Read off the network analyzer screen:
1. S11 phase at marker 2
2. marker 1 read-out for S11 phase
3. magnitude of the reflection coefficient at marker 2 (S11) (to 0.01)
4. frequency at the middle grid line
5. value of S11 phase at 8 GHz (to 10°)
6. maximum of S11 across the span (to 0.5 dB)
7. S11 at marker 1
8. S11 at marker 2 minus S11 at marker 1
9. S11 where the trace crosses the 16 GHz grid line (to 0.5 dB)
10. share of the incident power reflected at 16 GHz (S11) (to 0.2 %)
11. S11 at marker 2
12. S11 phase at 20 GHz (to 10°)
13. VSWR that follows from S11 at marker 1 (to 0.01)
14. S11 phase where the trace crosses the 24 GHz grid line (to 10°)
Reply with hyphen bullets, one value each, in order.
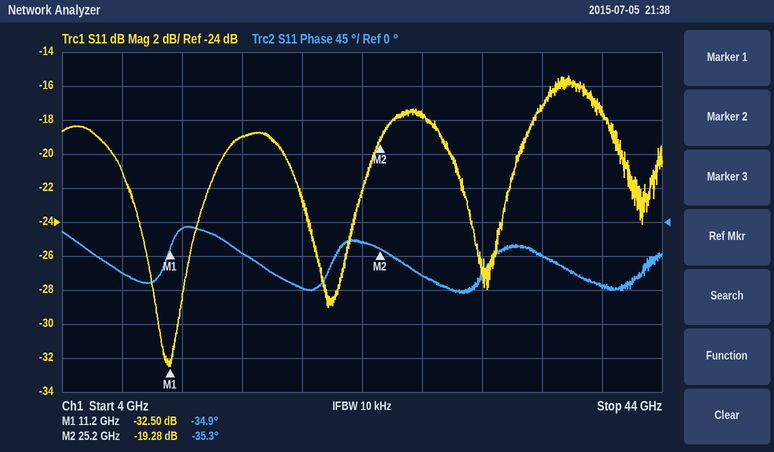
- -35.3°
- -34.9°
- 0.11
- 24 GHz
- -70°
- -15.5 dB
- -32.50 dB
- 13.22 dB
- -19.0 dB
- 1.2 %
- -19.28 dB
- -90°
- 1.05
- -30°
